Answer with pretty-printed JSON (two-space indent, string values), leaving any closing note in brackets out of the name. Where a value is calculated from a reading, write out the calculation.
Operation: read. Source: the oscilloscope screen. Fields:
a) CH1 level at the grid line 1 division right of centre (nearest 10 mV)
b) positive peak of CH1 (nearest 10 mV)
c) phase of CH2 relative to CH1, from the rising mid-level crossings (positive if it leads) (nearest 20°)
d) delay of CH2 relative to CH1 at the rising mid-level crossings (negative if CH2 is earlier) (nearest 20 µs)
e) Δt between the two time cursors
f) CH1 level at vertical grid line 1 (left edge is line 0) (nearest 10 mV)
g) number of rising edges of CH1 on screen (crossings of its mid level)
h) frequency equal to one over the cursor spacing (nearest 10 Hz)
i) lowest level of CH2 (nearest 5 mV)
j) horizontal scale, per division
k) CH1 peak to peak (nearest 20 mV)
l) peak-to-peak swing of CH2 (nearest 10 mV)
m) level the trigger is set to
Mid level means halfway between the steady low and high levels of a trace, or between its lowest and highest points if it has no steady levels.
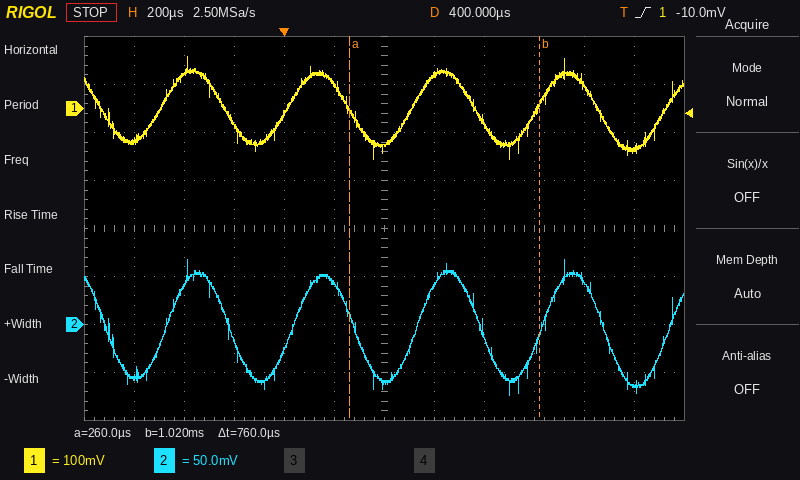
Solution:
{
  "CH1 level at the grid line 1 division right of centre": "70 mV",
  "positive peak of CH1": "110 mV",
  "phase of CH2 relative to CH1, from the rising mid-level crossings (positive if it leads)": "-20°",
  "delay of CH2 relative to CH1 at the rising mid-level crossings (negative if CH2 is earlier)": "+20 µs",
  "Δt between the two time cursors": "760 µs",
  "CH1 level at vertical grid line 1 (left edge is line 0)": "-60 mV",
  "number of rising edges of CH1 on screen": "5",
  "frequency equal to one over the cursor spacing": "1 / 760 µs ≈ 1.32 kHz",
  "lowest level of CH2": "-75 mV",
  "horizontal scale, per division": "200 µs",
  "CH1 peak to peak": "220 mV",
  "peak-to-peak swing of CH2": "140 mV",
  "level the trigger is set to": "-10.0 mV"
}
